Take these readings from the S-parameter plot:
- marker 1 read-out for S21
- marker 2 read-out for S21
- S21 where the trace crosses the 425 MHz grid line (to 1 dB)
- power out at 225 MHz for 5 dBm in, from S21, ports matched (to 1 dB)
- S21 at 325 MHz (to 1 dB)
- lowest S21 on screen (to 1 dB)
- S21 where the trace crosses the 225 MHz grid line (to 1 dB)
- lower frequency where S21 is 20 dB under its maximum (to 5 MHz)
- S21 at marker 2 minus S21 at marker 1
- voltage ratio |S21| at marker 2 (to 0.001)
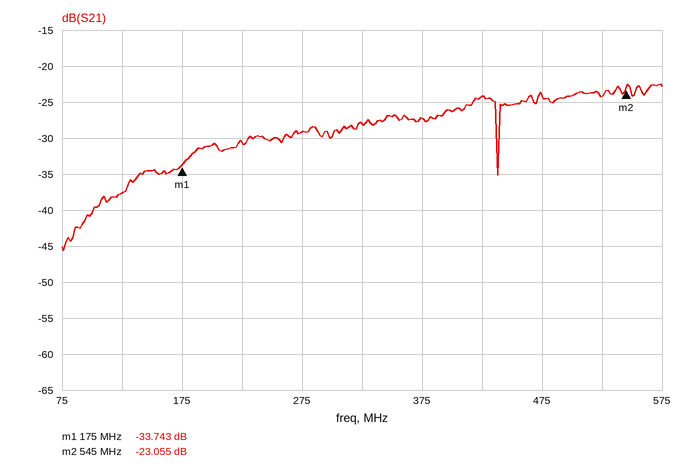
-33.743 dB
-23.055 dB
-24 dB
-26 dBm
-28 dB
-46 dB
-31 dB
85 MHz
10.688 dB
0.070
